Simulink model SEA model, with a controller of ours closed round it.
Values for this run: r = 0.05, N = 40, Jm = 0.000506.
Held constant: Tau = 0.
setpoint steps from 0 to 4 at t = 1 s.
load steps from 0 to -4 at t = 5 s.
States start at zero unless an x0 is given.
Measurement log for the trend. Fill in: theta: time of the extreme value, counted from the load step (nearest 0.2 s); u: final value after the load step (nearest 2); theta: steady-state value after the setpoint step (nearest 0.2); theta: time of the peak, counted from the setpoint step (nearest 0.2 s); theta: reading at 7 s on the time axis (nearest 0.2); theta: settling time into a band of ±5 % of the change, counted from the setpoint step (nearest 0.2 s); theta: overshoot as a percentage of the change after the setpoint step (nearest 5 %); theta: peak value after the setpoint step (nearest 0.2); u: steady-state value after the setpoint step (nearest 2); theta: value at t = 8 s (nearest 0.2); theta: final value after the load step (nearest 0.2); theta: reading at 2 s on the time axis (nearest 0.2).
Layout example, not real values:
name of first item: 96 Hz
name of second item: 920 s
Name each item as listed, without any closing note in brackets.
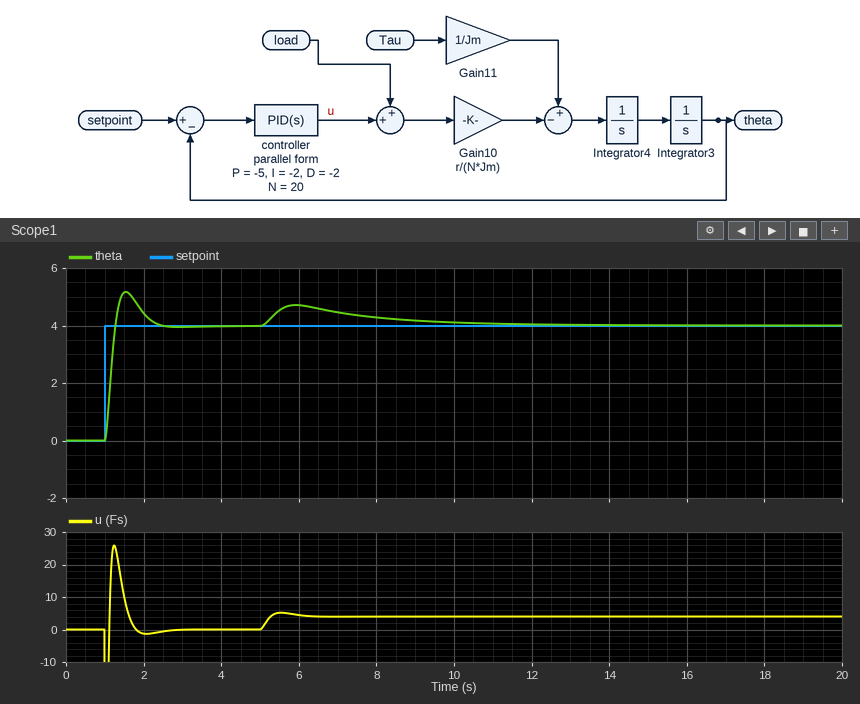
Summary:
theta: time of the extreme value, counted from the load step: 1.0 s
u: final value after the load step: 4
theta: steady-state value after the setpoint step: 4.0
theta: time of the peak, counted from the setpoint step: 0.6 s
theta: reading at 7 s on the time axis: 4.4
theta: settling time into a band of ±5 % of the change, counted from the setpoint step: 1.2 s
theta: overshoot as a percentage of the change after the setpoint step: 30 %
theta: peak value after the setpoint step: 5.2
u: steady-state value after the setpoint step: 0
theta: value at t = 8 s: 4.2
theta: final value after the load step: 4.0
theta: reading at 2 s on the time axis: 4.4
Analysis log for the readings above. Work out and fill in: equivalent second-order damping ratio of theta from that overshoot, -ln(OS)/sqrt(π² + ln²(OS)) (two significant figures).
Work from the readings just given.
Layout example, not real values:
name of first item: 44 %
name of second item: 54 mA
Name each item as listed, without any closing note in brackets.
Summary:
equivalent second-order damping ratio of theta from that overshoot, -ln(OS)/sqrt(π² + ln²(OS)): 0.36
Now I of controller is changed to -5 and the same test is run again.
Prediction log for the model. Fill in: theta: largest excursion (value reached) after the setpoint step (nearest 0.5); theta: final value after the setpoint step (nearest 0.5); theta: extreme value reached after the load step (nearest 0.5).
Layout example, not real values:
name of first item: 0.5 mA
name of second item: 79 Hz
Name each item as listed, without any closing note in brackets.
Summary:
theta: largest excursion (value reached) after the setpoint step: 5.5
theta: final value after the setpoint step: 4.0
theta: extreme value reached after the load step: 4.5
